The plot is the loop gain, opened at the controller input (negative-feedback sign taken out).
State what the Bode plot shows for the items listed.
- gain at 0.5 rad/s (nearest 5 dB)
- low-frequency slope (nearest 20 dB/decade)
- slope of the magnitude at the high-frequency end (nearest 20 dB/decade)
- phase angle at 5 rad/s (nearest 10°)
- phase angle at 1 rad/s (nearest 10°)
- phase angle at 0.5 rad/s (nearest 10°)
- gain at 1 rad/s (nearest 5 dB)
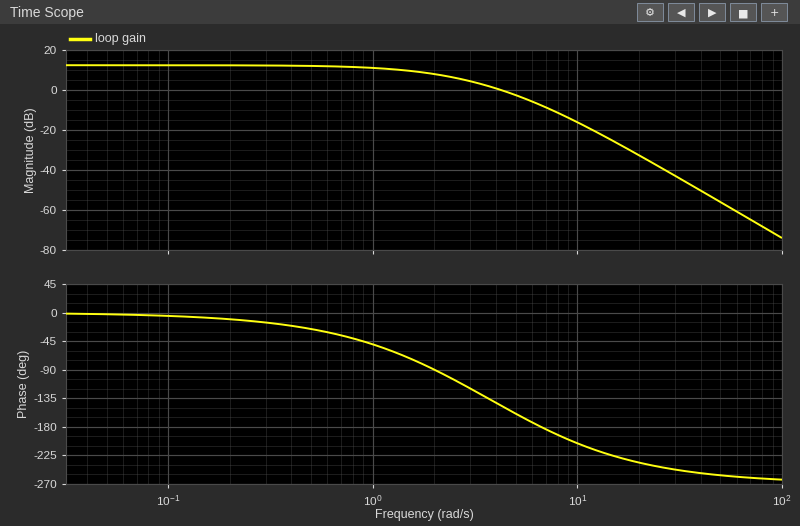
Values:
10 dB
0 dB/decade
-60 dB/decade
-160°
-50°
-30°
10 dB
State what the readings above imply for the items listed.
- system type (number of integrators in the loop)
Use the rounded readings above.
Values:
0
